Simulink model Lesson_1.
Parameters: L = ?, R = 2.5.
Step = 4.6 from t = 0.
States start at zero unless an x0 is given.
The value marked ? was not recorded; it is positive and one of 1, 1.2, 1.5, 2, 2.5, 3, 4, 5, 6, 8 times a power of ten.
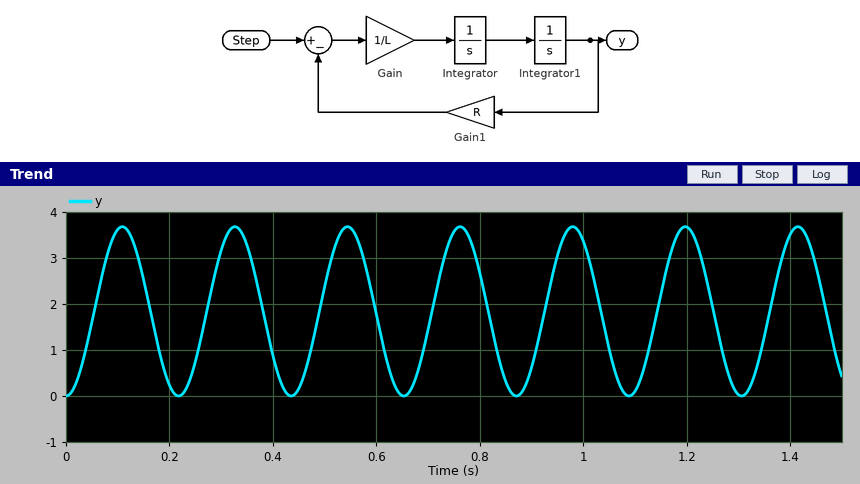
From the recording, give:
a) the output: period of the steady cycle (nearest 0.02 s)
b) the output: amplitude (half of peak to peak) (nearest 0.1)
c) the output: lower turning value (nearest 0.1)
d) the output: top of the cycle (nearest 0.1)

0.22 s
1.8
0.0
3.7
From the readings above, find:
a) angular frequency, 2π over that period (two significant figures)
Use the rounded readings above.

29 rad/s
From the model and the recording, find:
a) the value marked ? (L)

0.003
